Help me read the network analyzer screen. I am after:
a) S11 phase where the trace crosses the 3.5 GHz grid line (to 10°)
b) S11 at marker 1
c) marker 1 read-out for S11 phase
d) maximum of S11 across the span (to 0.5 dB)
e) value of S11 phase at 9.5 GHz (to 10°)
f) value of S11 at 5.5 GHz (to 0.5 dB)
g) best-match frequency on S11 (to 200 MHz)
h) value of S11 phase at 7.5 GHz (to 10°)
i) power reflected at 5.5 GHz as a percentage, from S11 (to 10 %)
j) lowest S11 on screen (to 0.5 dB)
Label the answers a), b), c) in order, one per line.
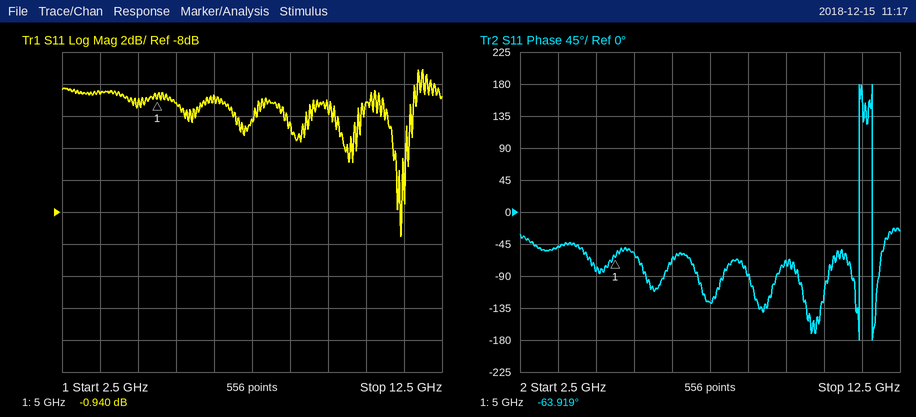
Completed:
a) -50°
b) -0.940 dB
c) -63.919°
d) 1.0 dB
e) -70°
f) -1.0 dB
g) 11.4 GHz
h) -130°
i) 80 %
j) -9.5 dB
